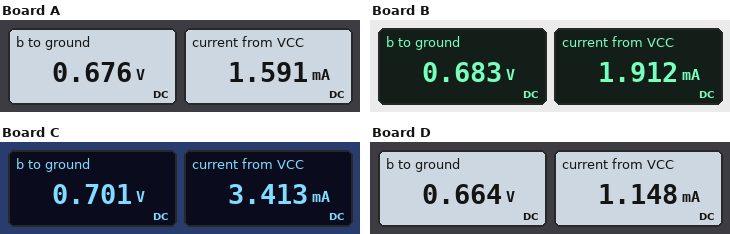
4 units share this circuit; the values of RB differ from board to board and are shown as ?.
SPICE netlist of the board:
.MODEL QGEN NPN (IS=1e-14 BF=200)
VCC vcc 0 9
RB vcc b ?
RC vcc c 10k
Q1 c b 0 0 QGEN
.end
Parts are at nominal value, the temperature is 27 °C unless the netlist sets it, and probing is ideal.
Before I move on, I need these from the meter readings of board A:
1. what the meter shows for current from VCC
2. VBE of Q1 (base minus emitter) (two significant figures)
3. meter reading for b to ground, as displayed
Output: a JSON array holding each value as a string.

["1.591 mA", "680 mV", "0.676 V"]
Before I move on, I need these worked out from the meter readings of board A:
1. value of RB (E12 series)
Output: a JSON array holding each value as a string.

["12 kΩ"]
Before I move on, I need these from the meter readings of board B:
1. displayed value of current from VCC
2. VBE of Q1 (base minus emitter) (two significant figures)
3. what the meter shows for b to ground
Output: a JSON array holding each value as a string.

["1.912 mA", "680 mV", "0.683 V"]
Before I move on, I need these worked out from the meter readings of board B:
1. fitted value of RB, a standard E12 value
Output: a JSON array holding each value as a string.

["8.2 kΩ"]
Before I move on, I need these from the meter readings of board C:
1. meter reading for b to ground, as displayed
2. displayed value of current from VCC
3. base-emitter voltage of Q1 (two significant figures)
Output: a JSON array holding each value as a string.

["0.701 V", "3.413 mA", "700 mV"]
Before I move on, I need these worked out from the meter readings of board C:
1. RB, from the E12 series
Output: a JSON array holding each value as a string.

["3.3 kΩ"]
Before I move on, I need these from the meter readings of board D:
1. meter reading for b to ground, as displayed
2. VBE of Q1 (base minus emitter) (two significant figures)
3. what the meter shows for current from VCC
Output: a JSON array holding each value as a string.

["0.664 V", "660 mV", "1.148 mA"]
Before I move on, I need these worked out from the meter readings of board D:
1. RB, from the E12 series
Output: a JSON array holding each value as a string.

["33 kΩ"]
